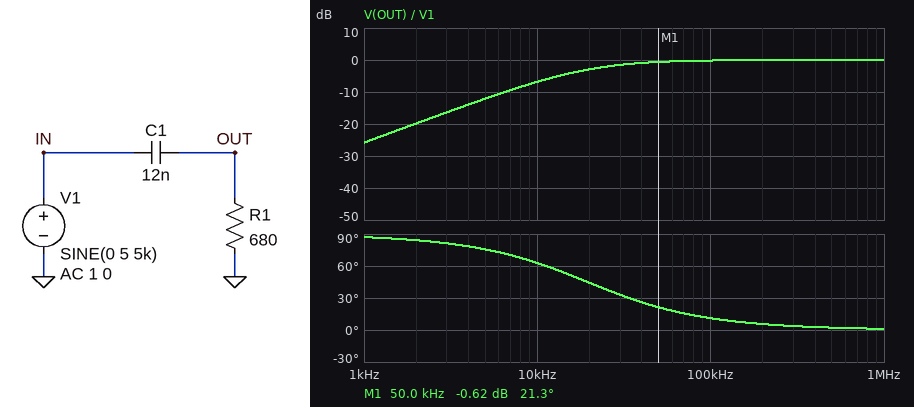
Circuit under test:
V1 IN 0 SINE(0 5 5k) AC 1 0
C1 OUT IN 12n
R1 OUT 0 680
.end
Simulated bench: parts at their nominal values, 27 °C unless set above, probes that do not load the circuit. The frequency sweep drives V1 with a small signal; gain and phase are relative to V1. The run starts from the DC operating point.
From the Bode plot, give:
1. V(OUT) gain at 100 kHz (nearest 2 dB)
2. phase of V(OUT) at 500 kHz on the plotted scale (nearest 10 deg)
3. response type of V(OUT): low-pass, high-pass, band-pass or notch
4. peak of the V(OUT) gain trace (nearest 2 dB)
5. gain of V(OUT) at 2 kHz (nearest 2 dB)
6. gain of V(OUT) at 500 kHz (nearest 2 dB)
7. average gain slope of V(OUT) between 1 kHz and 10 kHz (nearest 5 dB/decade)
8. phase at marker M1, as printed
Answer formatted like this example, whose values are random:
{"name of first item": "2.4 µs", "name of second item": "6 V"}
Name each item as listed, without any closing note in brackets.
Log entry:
{"V(OUT) gain at 100 kHz": "0 dB", "phase of V(OUT) at 500 kHz on the plotted scale": "0 deg", "response type of V(OUT): low-pass, high-pass, band-pass or notch": "high-pass", "peak of the V(OUT) gain trace": "0 dB", "gain of V(OUT) at 2 kHz": "-20 dB", "gain of V(OUT) at 500 kHz": "0 dB", "average gain slope of V(OUT) between 1 kHz and 10 kHz": "20 dB/decade", "phase at marker M1, as printed": "21.3 deg"}
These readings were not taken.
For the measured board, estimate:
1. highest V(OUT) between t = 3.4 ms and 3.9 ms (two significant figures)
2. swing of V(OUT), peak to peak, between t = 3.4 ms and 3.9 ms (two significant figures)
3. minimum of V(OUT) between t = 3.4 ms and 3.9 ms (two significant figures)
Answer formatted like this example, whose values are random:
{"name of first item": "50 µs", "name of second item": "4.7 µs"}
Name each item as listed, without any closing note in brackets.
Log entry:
{"highest V(OUT) between t = 3.4 ms and 3.9 ms": "1.2 V", "swing of V(OUT), peak to peak, between t = 3.4 ms and 3.9 ms": "2.5 V", "minimum of V(OUT) between t = 3.4 ms and 3.9 ms": "-1.2 V"}
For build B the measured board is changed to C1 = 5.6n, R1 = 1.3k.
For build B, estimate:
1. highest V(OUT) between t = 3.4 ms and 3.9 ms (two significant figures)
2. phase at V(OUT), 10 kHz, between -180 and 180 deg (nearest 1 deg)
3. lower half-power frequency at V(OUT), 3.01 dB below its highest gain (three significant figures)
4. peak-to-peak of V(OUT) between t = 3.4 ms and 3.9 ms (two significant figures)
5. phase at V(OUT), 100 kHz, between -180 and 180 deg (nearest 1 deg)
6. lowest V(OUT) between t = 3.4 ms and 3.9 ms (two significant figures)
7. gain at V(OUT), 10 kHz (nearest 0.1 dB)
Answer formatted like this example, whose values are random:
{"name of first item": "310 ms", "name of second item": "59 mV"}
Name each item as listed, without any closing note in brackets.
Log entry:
{"highest V(OUT) between t = 3.4 ms and 3.9 ms": "1.1 V", "phase at V(OUT), 10 kHz, between -180 and 180 deg": "65 deg", "lower half-power frequency at V(OUT), 3.01 dB below its highest gain": "21.9 kHz", "peak-to-peak of V(OUT) between t = 3.4 ms and 3.9 ms": "2.2 V", "phase at V(OUT), 100 kHz, between -180 and 180 deg": "12 deg", "lowest V(OUT) between t = 3.4 ms and 3.9 ms": "-1.1 V", "gain at V(OUT), 10 kHz": "-7.6 dB"}
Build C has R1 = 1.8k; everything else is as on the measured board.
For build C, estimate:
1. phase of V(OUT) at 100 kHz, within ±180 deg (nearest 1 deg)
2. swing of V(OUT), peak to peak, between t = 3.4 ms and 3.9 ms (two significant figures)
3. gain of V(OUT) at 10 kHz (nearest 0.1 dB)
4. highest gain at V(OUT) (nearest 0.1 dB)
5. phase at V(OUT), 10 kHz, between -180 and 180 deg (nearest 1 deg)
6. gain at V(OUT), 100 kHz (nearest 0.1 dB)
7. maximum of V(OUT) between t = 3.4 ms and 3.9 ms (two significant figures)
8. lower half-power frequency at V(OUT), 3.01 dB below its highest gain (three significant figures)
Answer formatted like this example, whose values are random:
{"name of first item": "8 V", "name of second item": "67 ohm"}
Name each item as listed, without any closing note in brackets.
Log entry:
{"phase of V(OUT) at 100 kHz, within ±180 deg": "4 deg", "swing of V(OUT), peak to peak, between t = 3.4 ms and 3.9 ms": "5.6 V", "gain of V(OUT) at 10 kHz": "-1.9 dB", "highest gain at V(OUT)": "0 dB", "phase at V(OUT), 10 kHz, between -180 and 180 deg": "36 deg", "gain at V(OUT), 100 kHz": "0 dB", "maximum of V(OUT) between t = 3.4 ms and 3.9 ms": "2.8 V", "lower half-power frequency at V(OUT), 3.01 dB below its highest gain": "7.37 kHz"}
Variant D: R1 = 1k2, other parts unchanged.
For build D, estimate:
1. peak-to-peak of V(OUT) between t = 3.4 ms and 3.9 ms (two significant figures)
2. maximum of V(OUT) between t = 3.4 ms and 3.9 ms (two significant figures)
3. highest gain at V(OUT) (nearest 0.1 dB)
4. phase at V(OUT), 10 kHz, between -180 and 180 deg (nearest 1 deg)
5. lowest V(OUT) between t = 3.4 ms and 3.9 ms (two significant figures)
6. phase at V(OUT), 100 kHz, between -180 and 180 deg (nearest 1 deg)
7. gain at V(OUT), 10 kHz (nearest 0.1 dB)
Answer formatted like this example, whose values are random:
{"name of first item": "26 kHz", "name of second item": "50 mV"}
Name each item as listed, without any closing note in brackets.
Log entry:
{"peak-to-peak of V(OUT) between t = 3.4 ms and 3.9 ms": "4.1 V", "maximum of V(OUT) between t = 3.4 ms and 3.9 ms": "2.1 V", "highest gain at V(OUT)": "0 dB", "phase at V(OUT), 10 kHz, between -180 and 180 deg": "48 deg", "lowest V(OUT) between t = 3.4 ms and 3.9 ms": "-2.1 V", "phase at V(OUT), 100 kHz, between -180 and 180 deg": "6 deg", "gain at V(OUT), 10 kHz": "-3.5 dB"}
